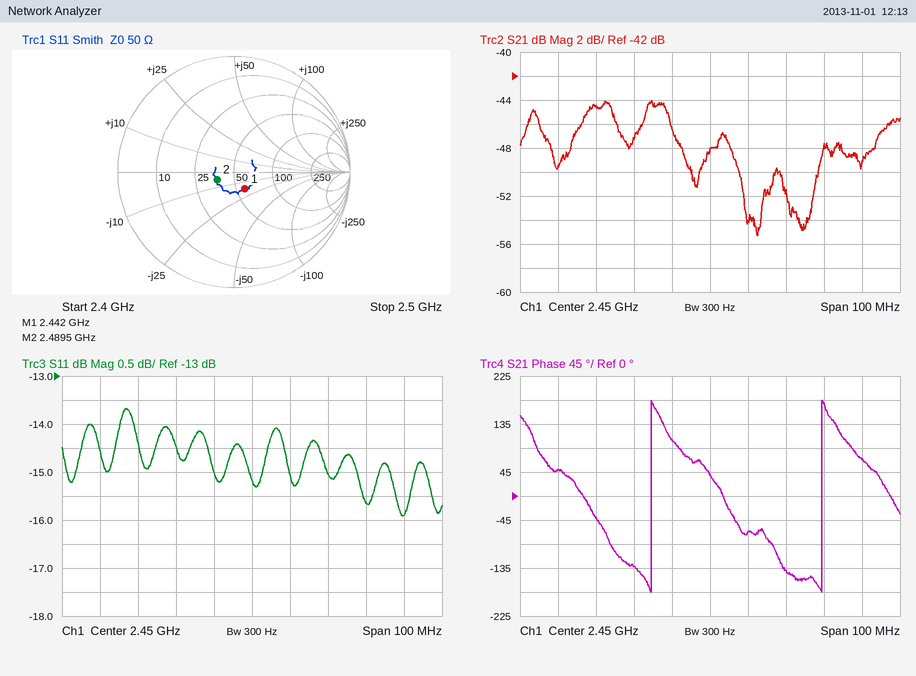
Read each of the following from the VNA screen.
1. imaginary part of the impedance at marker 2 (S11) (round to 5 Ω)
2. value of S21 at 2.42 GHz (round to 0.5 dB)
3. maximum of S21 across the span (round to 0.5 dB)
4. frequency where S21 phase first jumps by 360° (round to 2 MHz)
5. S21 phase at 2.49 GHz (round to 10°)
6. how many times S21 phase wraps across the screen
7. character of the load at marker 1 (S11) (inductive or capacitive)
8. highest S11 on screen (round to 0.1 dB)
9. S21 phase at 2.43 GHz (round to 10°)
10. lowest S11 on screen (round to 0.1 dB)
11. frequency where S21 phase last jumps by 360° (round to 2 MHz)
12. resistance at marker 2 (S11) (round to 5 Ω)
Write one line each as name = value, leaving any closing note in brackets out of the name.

imaginary part of the impedance at marker 2 (S11) = -5 Ω
value of S21 at 2.42 GHz = -44.5 dB
maximum of S21 across the span = -44.0 dB
frequency where S21 phase first jumps by 360° = 2.434 GHz
S21 phase at 2.49 GHz = 70°
how many times S21 phase wraps across the screen = 2
character of the load at marker 1 (S11) = capacitive
highest S11 on screen = -13.7 dB
S21 phase at 2.43 GHz = -130°
lowest S11 on screen = -15.9 dB
frequency where S21 phase last jumps by 360° = 2.480 GHz
resistance at marker 2 (S11) = 35 Ω
